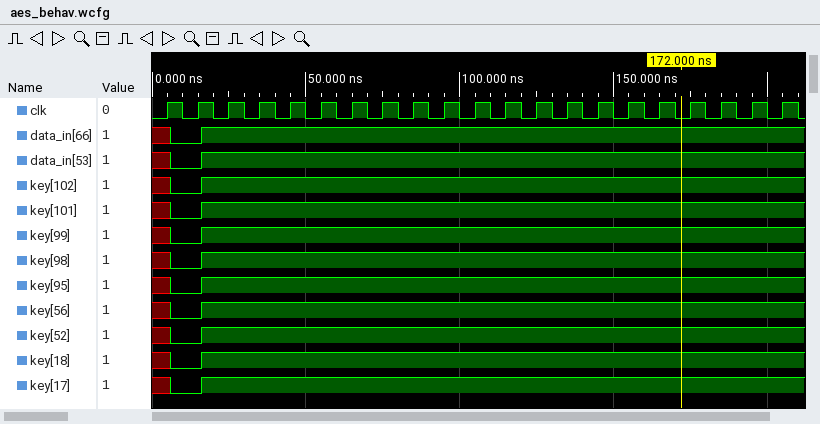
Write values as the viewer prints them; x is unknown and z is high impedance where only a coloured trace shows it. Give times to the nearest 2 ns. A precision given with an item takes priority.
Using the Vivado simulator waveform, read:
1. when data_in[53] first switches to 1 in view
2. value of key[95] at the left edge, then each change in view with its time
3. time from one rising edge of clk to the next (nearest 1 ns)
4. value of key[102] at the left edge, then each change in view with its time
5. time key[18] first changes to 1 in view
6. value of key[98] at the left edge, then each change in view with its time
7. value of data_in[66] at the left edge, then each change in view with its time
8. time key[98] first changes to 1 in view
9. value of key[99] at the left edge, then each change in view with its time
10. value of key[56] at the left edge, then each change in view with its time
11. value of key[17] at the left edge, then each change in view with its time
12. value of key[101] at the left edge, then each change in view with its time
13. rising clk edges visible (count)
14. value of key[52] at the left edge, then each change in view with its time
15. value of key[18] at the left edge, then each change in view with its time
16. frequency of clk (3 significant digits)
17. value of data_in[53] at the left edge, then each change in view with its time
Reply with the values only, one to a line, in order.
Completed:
16 ns
x, 0 at 6 ns, 1 at 16 ns
10 ns
x, 0 at 6 ns, 1 at 16 ns
16 ns
x, 0 at 6 ns, 1 at 16 ns
x, 0 at 6 ns, 1 at 16 ns
16 ns
x, 0 at 6 ns, 1 at 16 ns
x, 0 at 6 ns, 1 at 16 ns
x, 0 at 6 ns, 1 at 16 ns
x, 0 at 6 ns, 1 at 16 ns
21
x, 0 at 6 ns, 1 at 16 ns
x, 0 at 6 ns, 1 at 16 ns
100 MHz
x, 0 at 6 ns, 1 at 16 ns
